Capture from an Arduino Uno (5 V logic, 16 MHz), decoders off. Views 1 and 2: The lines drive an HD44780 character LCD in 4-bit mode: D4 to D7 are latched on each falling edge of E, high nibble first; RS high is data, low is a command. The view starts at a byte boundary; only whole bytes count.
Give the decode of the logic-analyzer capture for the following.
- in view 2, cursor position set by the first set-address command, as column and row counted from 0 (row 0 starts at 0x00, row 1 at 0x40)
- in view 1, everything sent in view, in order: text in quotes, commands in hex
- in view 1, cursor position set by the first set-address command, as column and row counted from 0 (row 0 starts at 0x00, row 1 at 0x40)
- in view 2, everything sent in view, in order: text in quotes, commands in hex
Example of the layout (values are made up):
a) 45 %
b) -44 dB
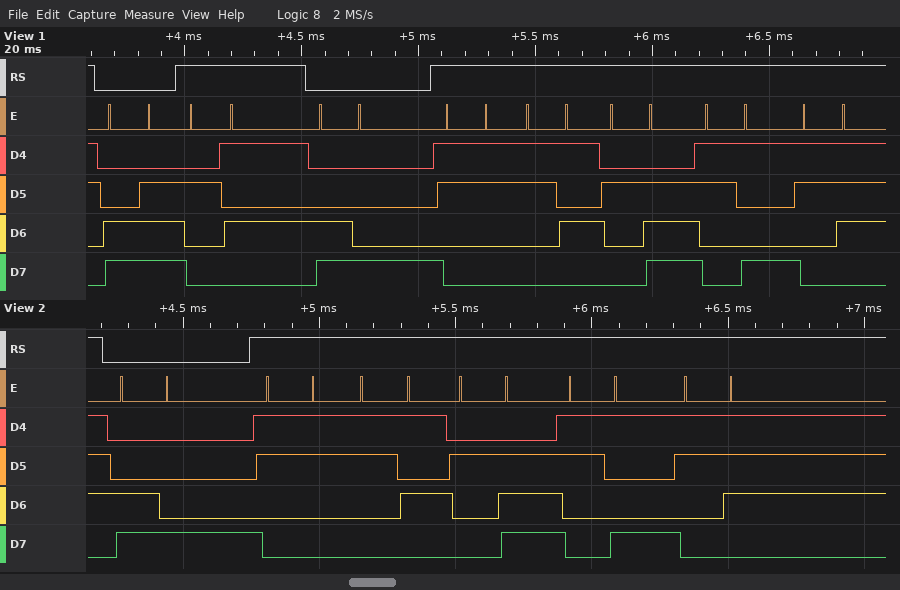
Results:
a) column 8, row 1
b) 0xCE "%" 0xC8 "35.97"
c) column 14, row 1
d) 0xC8 "35.97"
